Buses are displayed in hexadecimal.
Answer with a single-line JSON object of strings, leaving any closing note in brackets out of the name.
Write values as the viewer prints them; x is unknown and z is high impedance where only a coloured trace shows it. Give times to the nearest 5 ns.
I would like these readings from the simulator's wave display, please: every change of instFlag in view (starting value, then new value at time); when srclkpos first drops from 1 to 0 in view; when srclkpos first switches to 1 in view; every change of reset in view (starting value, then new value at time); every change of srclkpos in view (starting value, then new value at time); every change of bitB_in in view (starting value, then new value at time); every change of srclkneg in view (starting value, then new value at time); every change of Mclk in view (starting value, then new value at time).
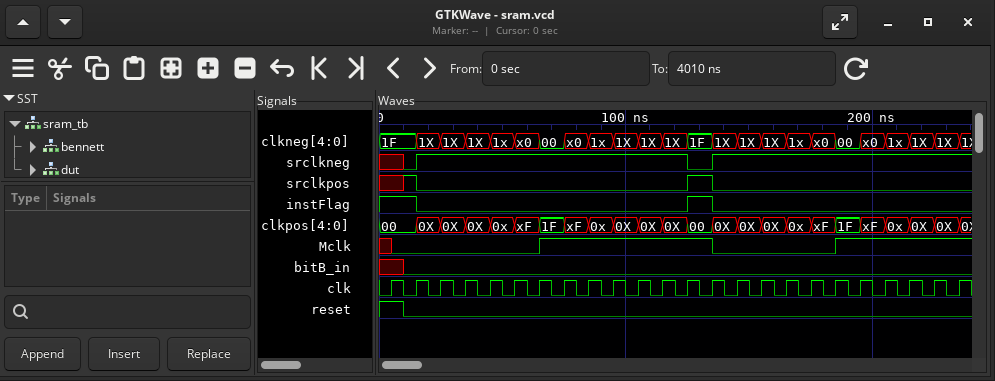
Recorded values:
{"every change of instFlag in view": "1, 0 at 15 ns, 1 at 125 ns, 0 at 135 ns", "when srclkpos first drops from 1 to 0 in view": "15 ns", "when srclkpos first switches to 1 in view": "10 ns", "every change of reset in view": "1, 0 at 10 ns", "every change of srclkpos in view": "x, 1 at 10 ns, 0 at 15 ns, 1 at 125 ns, 0 at 135 ns", "every change of bitB_in in view": "x, 0 at 10 ns", "every change of srclkneg in view": "x, 0 at 10 ns, 1 at 15 ns, 0 at 125 ns, 1 at 135 ns", "every change of Mclk in view": "x, 0 at 5 ns, 1 at 65 ns, 0 at 135 ns, 1 at 185 ns"}
